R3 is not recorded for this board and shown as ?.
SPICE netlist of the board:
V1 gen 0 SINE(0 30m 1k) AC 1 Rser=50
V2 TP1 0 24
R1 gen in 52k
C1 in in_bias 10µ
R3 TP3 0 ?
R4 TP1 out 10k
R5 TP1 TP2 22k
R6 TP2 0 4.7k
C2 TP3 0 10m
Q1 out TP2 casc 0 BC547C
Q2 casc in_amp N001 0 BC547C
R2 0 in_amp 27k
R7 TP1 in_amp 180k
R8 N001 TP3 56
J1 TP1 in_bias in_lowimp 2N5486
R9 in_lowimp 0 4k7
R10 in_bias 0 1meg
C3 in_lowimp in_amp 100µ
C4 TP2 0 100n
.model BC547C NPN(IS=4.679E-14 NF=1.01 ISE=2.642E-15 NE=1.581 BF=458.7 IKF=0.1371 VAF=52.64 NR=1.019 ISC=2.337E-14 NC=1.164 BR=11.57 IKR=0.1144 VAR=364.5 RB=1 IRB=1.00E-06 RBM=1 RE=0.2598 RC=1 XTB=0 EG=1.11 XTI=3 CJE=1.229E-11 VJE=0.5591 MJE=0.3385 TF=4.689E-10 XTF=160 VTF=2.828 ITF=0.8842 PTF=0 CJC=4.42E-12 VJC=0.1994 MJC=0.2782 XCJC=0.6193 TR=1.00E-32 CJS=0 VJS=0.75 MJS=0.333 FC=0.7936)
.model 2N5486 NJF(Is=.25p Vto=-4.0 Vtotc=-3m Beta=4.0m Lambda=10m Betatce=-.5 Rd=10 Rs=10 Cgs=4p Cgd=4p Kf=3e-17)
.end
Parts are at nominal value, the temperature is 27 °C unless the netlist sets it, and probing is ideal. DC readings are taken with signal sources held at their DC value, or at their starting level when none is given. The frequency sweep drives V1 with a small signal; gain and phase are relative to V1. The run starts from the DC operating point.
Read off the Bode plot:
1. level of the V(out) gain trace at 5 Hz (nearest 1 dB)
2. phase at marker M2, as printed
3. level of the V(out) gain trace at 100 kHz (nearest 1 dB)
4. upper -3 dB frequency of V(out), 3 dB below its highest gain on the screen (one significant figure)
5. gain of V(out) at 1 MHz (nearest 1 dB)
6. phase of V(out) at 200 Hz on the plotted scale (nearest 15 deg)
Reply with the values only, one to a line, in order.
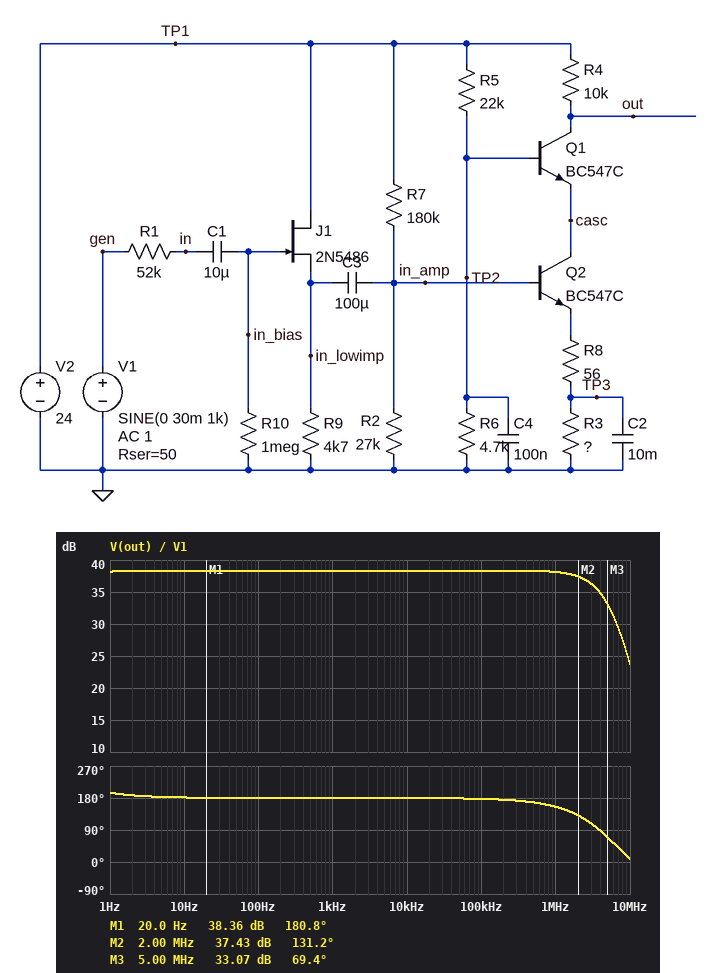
38 dB
131.2 deg
38 dB
4 MHz
38 dB
180 deg
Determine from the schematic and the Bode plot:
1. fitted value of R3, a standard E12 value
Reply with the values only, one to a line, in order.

4.7 kΩ
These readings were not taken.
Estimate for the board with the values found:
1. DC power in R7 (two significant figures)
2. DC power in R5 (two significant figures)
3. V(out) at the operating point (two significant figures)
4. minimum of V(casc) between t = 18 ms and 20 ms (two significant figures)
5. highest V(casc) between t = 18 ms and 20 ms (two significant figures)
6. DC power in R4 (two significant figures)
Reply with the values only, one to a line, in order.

2.4 mW
18 mW
19 V
3.6 V
3.6 V
2.7 mW
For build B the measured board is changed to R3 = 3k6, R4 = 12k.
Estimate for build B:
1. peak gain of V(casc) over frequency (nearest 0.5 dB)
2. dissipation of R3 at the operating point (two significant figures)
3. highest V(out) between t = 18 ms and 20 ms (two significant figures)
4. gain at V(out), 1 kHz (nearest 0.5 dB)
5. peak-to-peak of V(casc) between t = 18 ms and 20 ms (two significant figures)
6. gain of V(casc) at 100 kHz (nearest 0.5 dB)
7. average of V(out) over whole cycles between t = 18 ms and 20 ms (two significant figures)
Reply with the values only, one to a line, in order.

-6.5 dB
1.7 mW
19 V
41.0 dB
25 mV
-8.0 dB
16 V
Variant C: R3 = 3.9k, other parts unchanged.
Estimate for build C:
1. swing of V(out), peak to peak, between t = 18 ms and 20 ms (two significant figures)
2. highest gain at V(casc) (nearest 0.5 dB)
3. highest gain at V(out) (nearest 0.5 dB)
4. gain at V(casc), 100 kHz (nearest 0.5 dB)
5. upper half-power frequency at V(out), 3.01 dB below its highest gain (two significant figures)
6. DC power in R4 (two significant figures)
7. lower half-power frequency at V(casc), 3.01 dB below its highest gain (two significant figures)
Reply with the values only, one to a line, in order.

5.3 V
-6.5 dB
39.0 dB
-7.5 dB
3.6 MHz
3.9 mW
230 mHz
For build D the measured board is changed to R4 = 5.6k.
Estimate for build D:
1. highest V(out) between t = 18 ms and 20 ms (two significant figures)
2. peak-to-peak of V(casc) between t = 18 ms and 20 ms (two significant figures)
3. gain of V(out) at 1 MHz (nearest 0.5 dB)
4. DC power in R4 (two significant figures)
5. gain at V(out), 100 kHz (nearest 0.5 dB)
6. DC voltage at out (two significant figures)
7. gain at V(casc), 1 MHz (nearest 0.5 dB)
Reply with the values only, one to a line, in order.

22 V
27 mV
33.0 dB
1.5 mW
33.5 dB
21 V
-7.5 dB
